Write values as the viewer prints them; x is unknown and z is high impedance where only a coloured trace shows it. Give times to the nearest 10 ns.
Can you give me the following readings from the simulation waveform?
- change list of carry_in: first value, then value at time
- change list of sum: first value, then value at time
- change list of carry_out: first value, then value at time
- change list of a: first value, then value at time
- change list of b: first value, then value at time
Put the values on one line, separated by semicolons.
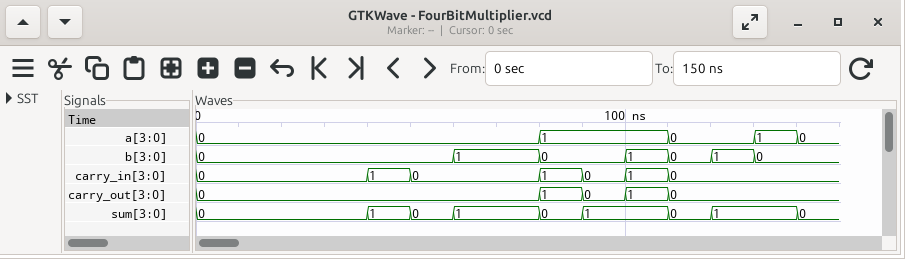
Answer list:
0, 1 at 40 ns, 0 at 50 ns, 1 at 80 ns, 0 at 90 ns, 1 at 100 ns, 0 at 110 ns; 0, 1 at 40 ns, 0 at 50 ns, 1 at 60 ns, 0 at 80 ns, 1 at 90 ns, 0 at 110 ns, 1 at 120 ns, 0 at 140 ns; 0, 1 at 80 ns, 0 at 90 ns, 1 at 100 ns, 0 at 110 ns; 0, 1 at 80 ns, 0 at 110 ns, 1 at 130 ns, 0 at 140 ns; 0, 1 at 60 ns, 0 at 80 ns, 1 at 100 ns, 0 at 110 ns, 1 at 120 ns, 0 at 130 ns
